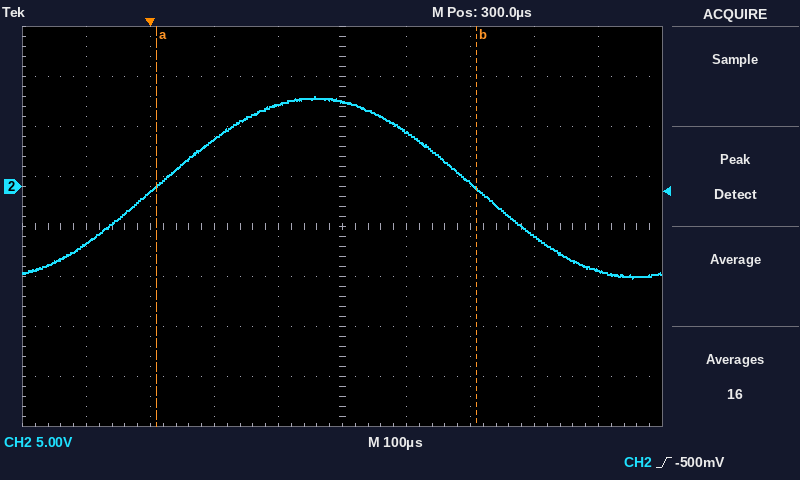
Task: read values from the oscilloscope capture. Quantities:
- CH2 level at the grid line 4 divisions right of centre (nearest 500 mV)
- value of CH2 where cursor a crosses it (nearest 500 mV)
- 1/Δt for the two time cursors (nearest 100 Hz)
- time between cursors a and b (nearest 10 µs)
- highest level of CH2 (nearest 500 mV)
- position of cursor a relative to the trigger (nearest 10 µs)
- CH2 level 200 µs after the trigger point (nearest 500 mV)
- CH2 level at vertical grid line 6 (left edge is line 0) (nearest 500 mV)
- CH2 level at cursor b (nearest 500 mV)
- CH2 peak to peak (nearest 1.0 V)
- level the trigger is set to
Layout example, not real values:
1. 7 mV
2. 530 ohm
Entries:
1. -8.5 V
2. 0.0 V
3. 2.0 kHz
4. 500 µs
5. 9.0 V
6. +10 µs
7. 8.0 V
8. 5.5 V
9. 0.0 V
10. 18.0 V
11. -500 mV
